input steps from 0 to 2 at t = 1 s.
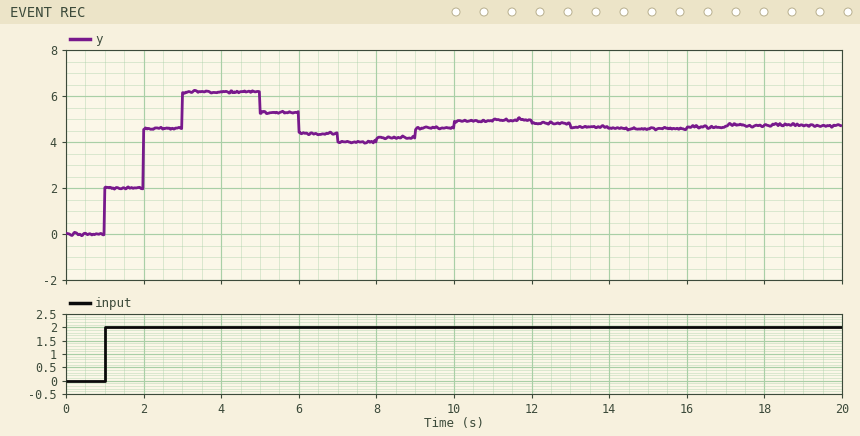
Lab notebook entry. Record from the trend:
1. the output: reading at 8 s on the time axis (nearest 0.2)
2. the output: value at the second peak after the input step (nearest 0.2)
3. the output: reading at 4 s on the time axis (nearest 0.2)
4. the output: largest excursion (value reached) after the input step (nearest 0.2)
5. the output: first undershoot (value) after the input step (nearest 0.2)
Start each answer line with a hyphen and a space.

- 4.2
- 5.0
- 6.2
- 6.2
- 4.0
